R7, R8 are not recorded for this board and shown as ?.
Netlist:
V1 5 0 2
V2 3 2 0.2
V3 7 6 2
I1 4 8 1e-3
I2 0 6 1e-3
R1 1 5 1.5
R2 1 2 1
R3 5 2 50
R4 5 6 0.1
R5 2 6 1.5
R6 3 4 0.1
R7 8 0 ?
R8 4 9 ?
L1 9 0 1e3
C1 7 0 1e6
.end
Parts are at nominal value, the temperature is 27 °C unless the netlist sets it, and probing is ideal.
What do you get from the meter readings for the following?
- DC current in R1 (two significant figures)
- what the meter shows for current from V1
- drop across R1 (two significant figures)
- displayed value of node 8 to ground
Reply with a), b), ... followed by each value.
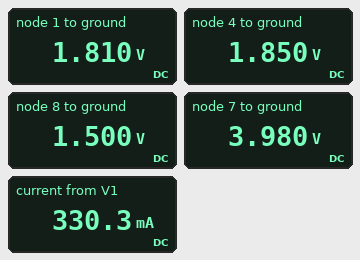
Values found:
a) 130 mA
b) 330.3 mA
c) 190 mV
d) 1.500 V
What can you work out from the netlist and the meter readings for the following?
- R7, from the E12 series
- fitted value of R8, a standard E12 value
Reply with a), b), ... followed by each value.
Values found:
a) 1.5 kΩ
b) 5.6 Ω
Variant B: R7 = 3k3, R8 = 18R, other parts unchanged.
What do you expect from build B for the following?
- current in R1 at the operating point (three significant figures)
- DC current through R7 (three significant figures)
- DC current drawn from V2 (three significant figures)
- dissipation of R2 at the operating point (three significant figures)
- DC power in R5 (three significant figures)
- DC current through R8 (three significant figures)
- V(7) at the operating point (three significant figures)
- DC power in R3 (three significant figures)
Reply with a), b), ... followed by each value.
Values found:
a) 44.5 mA
b) 1.00 mA
c) 116 mA
d) 1.98 mW
e) 7.27 mW
f) 115 mA
g) 3.99 V
h) 248 µW
